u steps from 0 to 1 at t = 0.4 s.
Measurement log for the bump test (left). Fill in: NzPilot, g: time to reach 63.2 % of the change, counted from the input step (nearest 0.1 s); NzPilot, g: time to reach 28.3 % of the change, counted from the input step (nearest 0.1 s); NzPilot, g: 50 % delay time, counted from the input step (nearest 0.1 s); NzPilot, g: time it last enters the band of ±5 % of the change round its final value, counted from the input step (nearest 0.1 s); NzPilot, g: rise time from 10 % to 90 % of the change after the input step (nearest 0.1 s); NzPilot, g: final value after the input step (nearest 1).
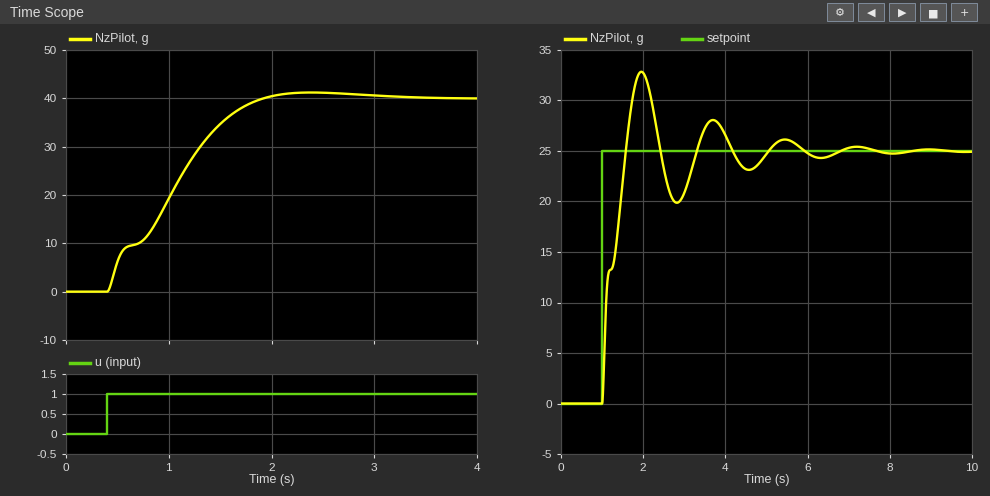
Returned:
0.8 s
0.4 s
0.6 s
1.3 s
1.1 s
40
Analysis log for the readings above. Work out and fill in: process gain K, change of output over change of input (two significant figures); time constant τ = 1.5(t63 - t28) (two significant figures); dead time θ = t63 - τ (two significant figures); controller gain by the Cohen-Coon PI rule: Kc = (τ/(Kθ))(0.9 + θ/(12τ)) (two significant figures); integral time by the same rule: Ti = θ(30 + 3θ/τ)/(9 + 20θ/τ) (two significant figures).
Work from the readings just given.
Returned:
40
0.60 s
0.20 s
0.070
0.40 s
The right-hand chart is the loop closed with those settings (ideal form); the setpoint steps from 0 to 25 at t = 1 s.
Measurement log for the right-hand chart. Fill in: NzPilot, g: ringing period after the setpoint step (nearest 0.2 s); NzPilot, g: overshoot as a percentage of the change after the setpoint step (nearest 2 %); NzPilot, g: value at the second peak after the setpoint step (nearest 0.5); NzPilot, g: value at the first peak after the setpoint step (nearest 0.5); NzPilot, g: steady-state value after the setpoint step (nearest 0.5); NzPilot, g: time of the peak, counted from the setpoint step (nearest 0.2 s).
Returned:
1.8 s
32 %
28.0
33.0
25.0
1.0 s
